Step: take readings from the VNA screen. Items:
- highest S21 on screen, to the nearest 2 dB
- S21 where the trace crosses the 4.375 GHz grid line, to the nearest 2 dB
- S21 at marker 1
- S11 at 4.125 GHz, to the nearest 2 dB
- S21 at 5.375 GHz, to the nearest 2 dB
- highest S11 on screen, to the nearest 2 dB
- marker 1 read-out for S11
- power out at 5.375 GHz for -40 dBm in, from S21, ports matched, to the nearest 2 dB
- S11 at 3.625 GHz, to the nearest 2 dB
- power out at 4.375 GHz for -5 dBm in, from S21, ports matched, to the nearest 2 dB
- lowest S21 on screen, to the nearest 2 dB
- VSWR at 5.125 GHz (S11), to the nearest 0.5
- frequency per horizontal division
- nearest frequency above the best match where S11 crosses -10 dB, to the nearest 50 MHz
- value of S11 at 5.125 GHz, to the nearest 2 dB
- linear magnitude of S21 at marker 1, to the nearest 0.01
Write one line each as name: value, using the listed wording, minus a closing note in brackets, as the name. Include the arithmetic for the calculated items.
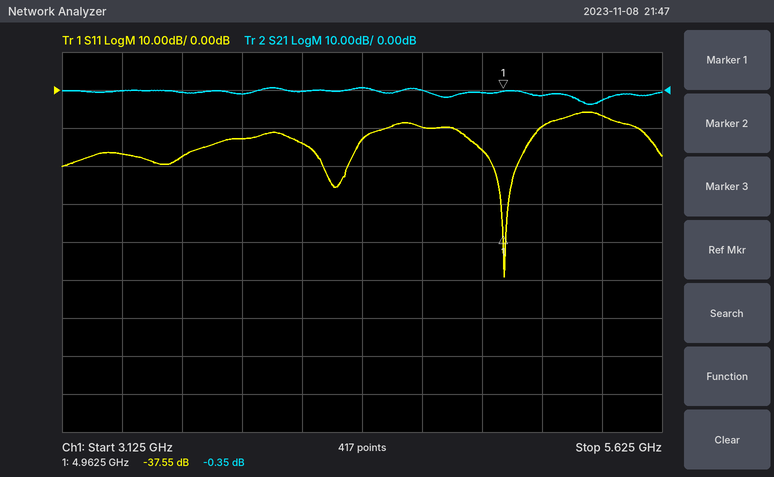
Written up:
highest S21 on screen, to the nearest 2 dB: 0 dB
S21 where the trace crosses the 4.375 GHz grid line, to the nearest 2 dB: 0 dB
S21 at marker 1: -0.35 dB
S11 at 4.125 GHz, to the nearest 2 dB: -14 dB
S21 at 5.375 GHz, to the nearest 2 dB: -2 dB
highest S11 on screen, to the nearest 2 dB: -6 dB
marker 1 read-out for S11: -37.55 dB
power out at 5.375 GHz for -40 dBm in, from S21, ports matched, to the nearest 2 dB: -40 dBm + (-2 dB) = -42 dBm
S11 at 3.625 GHz, to the nearest 2 dB: -18 dB
power out at 4.375 GHz for -5 dBm in, from S21, ports matched, to the nearest 2 dB: -5 dBm + (0 dB) = -4 dBm
lowest S21 on screen, to the nearest 2 dB: -4 dB
VSWR at 5.125 GHz (S11), to the nearest 0.5: |Γ| = 10^(-10/20) = 0.3162; VSWR = (1 + 0.3162)/(1 − 0.3162) ≈ 1.92, so 2.0 to the nearest 0.5
frequency per horizontal division: 250 MHz
nearest frequency above the best match where S11 crosses -10 dB, to the nearest 50 MHz: 5.10 GHz
value of S11 at 5.125 GHz, to the nearest 2 dB: -10 dB
linear magnitude of S21 at marker 1, to the nearest 0.01: 10^(-0.35/20) ≈ 0.96
